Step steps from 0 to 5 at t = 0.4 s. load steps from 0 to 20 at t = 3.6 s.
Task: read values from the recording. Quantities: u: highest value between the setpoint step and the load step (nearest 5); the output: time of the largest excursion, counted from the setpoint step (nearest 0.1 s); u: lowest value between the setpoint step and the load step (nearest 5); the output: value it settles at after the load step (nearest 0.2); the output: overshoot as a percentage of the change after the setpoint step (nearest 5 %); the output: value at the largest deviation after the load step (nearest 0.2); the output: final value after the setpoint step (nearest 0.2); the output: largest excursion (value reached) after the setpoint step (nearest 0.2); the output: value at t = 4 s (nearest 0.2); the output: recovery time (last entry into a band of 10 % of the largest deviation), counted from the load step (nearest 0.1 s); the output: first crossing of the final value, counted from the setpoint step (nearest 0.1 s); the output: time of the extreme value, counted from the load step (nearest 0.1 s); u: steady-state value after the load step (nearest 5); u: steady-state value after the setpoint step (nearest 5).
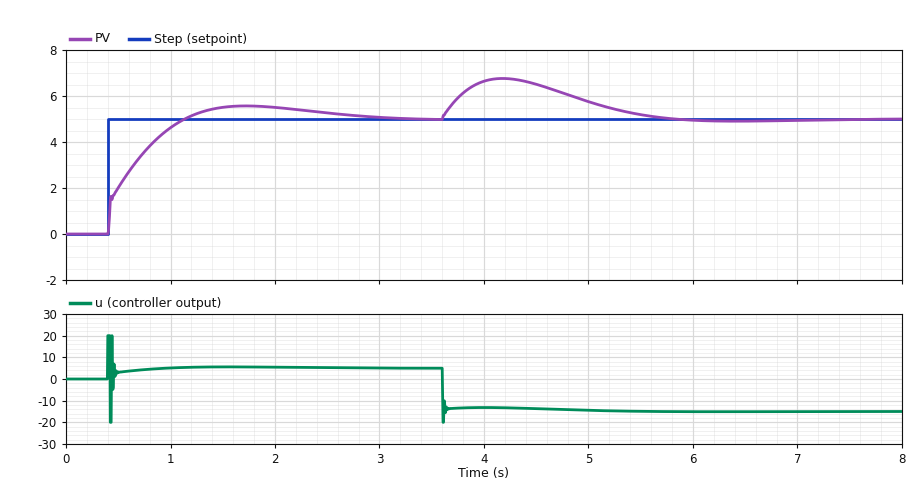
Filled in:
20
1.3 s
-20
5.0
10 %
6.8
5.0
5.6
6.6
1.9 s
0.7 s
0.6 s
-15
5
